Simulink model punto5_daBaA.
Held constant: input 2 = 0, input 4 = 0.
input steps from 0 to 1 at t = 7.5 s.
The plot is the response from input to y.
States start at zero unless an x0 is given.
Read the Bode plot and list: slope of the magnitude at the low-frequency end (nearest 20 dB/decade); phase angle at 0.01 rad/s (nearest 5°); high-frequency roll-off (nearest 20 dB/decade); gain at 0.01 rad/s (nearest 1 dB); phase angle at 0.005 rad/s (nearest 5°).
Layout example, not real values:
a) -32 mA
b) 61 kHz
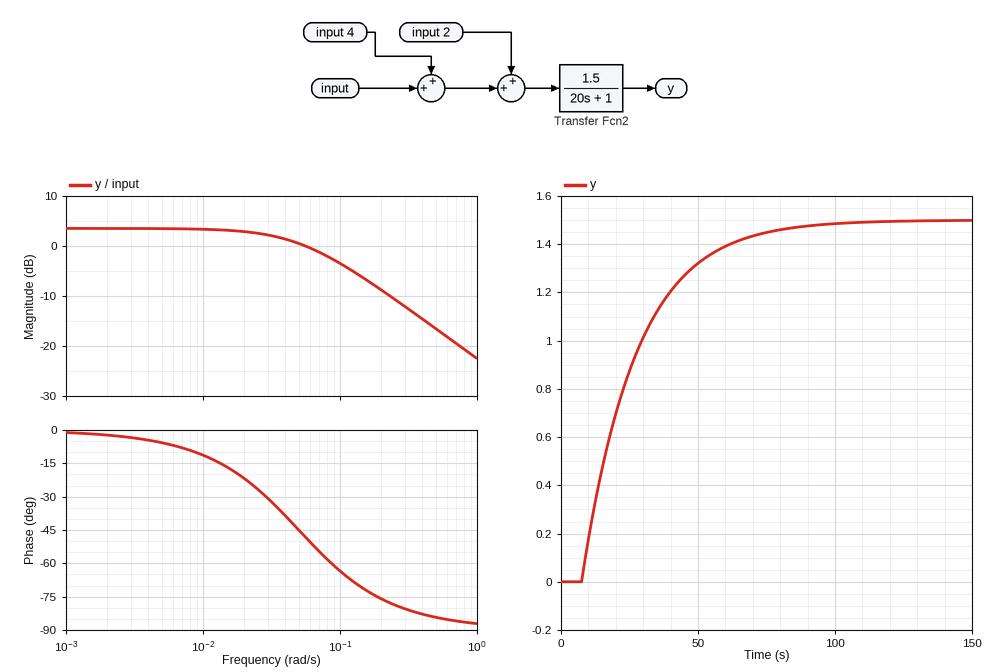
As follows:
a) 0 dB/decade
b) -10°
c) -20 dB/decade
d) 3 dB
e) -5°
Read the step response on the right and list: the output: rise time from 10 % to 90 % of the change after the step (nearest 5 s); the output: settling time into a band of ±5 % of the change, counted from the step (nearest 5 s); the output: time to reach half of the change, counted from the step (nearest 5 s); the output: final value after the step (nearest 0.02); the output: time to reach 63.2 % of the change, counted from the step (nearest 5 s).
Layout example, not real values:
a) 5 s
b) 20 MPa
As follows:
a) 45 s
b) 60 s
c) 15 s
d) 1.50
e) 20 s
